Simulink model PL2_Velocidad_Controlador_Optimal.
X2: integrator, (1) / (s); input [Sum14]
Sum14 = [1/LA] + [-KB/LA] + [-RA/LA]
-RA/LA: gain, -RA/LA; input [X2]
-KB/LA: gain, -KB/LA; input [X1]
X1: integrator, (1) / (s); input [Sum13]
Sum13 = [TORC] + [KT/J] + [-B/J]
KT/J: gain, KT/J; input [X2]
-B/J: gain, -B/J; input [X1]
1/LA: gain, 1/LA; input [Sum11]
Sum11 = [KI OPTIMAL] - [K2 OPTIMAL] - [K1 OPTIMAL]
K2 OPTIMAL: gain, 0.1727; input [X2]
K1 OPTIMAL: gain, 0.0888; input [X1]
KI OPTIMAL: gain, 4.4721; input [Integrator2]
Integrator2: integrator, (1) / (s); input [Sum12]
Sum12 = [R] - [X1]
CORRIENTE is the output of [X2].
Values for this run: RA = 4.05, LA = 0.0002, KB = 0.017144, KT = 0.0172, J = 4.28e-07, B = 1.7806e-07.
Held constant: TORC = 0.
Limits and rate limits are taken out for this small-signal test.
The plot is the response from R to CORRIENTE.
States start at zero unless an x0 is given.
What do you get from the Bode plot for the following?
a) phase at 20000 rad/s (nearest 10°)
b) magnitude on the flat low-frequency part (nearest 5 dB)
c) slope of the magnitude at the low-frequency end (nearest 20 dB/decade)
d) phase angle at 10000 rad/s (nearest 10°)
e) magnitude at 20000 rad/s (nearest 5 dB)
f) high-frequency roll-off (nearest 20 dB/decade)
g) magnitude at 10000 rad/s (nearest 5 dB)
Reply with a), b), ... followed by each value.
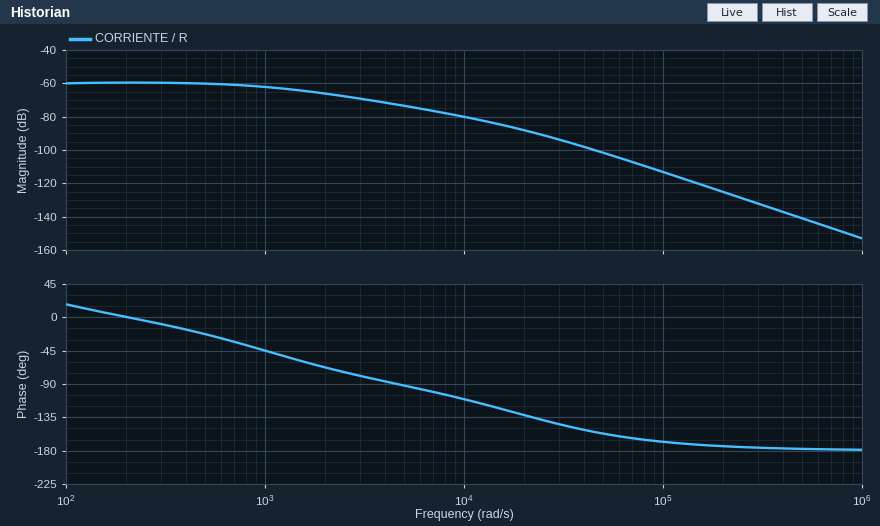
a) -130°
b) -60 dB
c) 0 dB/decade
d) -110°
e) -90 dB
f) -40 dB/decade
g) -80 dB
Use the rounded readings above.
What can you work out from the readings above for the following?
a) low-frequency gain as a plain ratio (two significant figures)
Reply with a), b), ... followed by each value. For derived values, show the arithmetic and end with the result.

a) 10^(-60 / 20) = 0.0010
